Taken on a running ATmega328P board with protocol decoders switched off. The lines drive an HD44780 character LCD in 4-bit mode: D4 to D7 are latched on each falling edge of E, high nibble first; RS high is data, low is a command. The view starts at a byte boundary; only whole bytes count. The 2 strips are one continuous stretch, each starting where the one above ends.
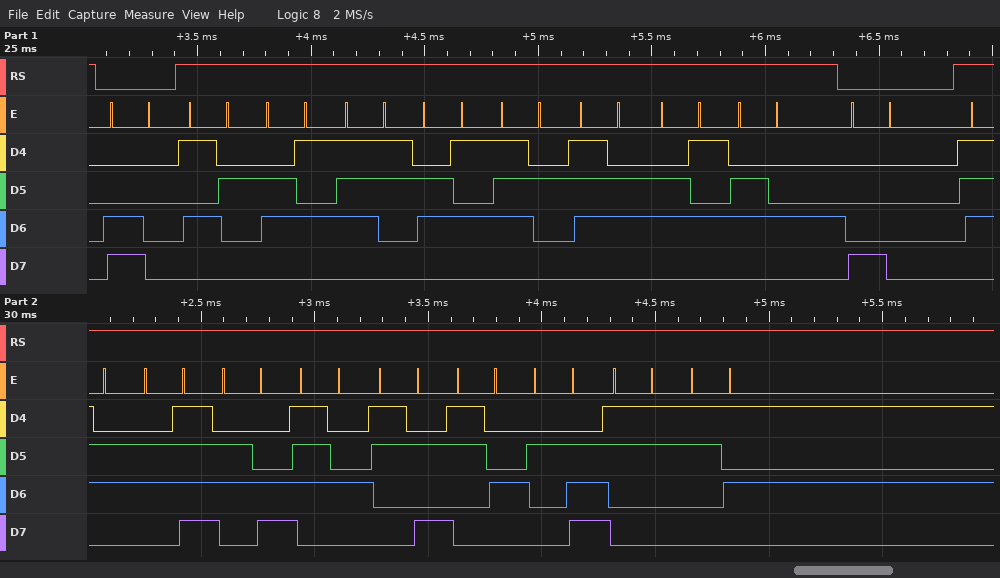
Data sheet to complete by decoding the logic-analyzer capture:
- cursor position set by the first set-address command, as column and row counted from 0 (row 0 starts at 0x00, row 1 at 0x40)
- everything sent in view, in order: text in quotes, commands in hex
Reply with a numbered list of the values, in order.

1. column 0, row 1
2. 0xC0 "Reserved" 0x80 "volt:4.35"
